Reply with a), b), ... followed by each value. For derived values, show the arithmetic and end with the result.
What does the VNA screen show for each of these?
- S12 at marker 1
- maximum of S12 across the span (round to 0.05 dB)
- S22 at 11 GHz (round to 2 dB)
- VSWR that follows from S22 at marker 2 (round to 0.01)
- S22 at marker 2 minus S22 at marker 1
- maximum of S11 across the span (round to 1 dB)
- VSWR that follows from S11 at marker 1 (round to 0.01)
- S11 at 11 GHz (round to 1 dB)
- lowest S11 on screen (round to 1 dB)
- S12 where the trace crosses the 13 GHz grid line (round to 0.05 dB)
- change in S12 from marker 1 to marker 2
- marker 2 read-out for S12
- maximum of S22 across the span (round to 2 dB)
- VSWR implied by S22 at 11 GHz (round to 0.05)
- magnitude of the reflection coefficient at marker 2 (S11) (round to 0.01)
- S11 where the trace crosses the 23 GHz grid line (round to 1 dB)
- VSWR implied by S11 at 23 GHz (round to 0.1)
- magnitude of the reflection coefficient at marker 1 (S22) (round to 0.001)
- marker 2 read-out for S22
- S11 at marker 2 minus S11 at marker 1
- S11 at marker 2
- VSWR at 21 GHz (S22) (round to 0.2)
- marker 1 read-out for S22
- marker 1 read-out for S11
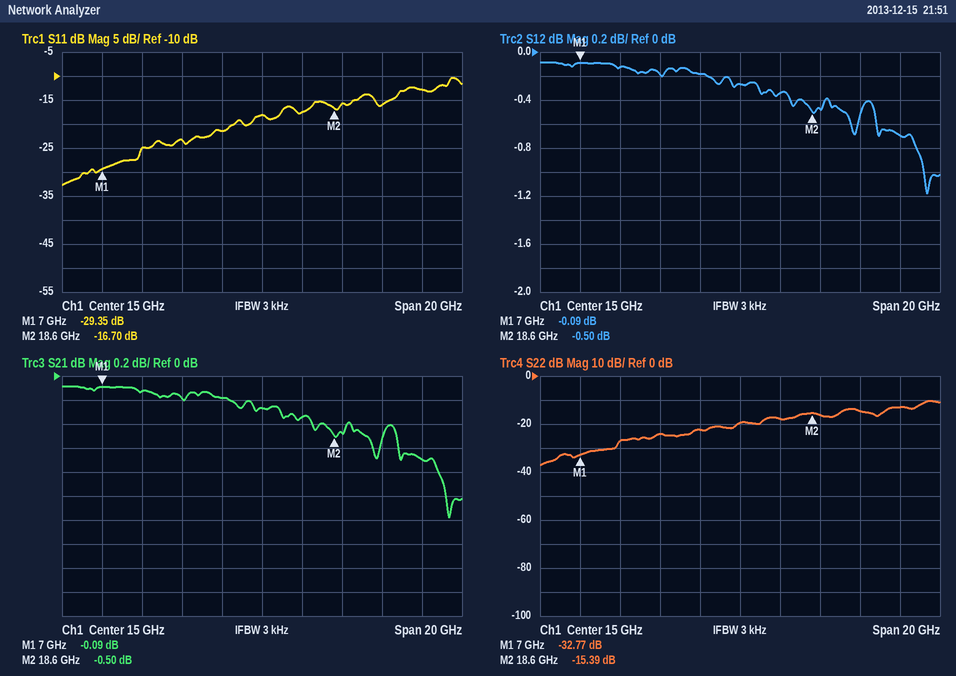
a) -0.09 dB
b) -0.10 dB
c) -24 dB
d) (1 + 0.1700)/(1 − 0.1700) ≈ 1.41
e) -15.39 − (-32.77) = 17.38 dB
f) -10 dB
g) (1 + 0.0341)/(1 − 0.0341) ≈ 1.07
h) -23 dB
i) -33 dB
j) -0.20 dB
k) -0.5 − (-0.09) = -0.41 dB
l) -0.50 dB
m) -10 dB
n) |Γ| = 10^(-24/20) = 0.0631; VSWR = (1 + 0.0631)/(1 − 0.0631) ≈ 1.13, so 1.15 to the nearest 0.05
o) 10^(-16.7/20) ≈ 0.15
p) -13 dB
q) |Γ| = 10^(-13/20) = 0.2239; VSWR = (1 + 0.2239)/(1 − 0.2239) ≈ 1.6
r) 10^(-32.77/20) ≈ 0.023
s) -15.39 dB
t) -16.7 − (-29.35) = 12.65 dB
u) -16.70 dB
v) |Γ| = 10^(-14/20) = 0.1995; VSWR = (1 + 0.1995)/(1 − 0.1995) ≈ 1.50, so 1.4 to the nearest 0.2
w) -32.77 dB
x) -29.35 dB
